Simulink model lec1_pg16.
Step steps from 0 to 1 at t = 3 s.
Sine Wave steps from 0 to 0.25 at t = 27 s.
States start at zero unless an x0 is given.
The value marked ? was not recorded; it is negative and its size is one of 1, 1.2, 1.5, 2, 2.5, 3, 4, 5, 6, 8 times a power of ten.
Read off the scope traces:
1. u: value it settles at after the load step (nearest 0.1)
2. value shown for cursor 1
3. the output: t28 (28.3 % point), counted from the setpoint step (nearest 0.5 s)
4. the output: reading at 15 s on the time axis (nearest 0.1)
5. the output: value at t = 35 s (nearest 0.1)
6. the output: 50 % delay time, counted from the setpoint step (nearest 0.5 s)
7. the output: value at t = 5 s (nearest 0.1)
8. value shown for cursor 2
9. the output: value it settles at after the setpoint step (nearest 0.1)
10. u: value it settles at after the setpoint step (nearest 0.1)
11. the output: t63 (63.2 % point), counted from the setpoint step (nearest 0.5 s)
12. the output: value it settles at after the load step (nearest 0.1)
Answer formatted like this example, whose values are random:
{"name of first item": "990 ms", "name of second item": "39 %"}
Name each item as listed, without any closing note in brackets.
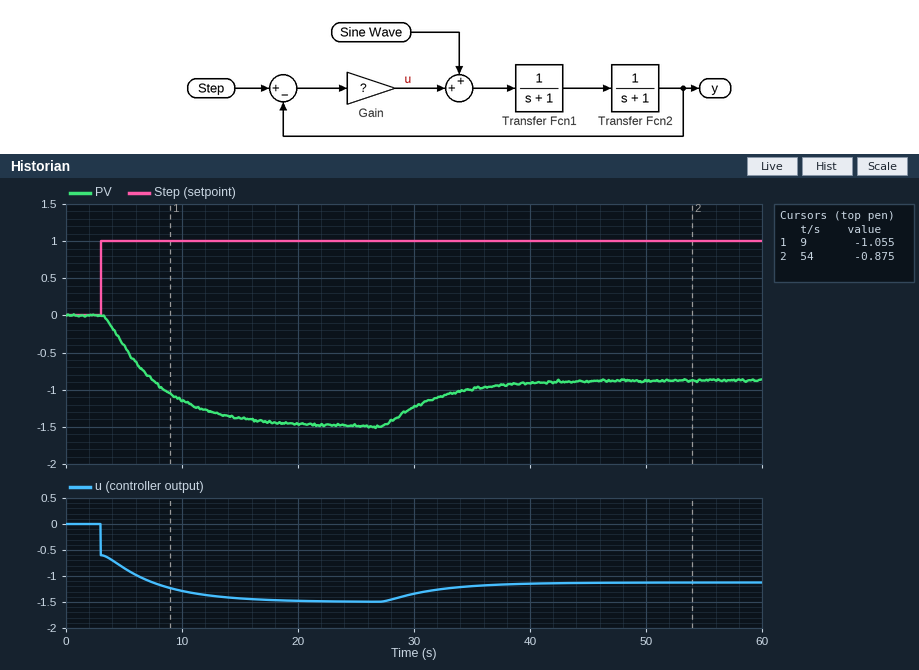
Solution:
{"u: value it settles at after the load step": "-1.1", "value shown for cursor 1": "-1.055", "the output: t28 (28.3 % point), counted from the setpoint step": "2.0 s", "the output: reading at 15 s on the time axis": "-1.4", "the output: value at t = 35 s": "-1.0", "the output: 50 % delay time, counted from the setpoint step": "3.5 s", "the output: value at t = 5 s": "-0.4", "value shown for cursor 2": "-0.875", "the output: value it settles at after the setpoint step": "-1.5", "u: value it settles at after the setpoint step": "-1.5", "the output: t63 (63.2 % point), counted from the setpoint step": "5.0 s", "the output: value it settles at after the load step": "-0.9"}
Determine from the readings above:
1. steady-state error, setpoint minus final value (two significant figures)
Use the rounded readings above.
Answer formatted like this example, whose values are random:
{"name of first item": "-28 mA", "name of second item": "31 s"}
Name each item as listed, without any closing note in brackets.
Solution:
{"steady-state error, setpoint minus final value": "2.5"}
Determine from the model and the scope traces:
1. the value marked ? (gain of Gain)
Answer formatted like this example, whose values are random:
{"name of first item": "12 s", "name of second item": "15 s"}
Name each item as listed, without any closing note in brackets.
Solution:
{"the value marked ?": "-0.6"}
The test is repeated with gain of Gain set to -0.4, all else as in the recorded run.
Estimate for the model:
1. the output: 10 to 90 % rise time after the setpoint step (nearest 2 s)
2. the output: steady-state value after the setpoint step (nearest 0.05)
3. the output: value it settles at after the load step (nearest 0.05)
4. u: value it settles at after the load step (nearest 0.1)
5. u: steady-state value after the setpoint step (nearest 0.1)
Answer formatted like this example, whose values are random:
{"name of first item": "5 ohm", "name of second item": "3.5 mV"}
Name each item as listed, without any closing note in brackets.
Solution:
{"the output: 10 to 90 % rise time after the setpoint step": "6 s", "the output: steady-state value after the setpoint step": "-0.65", "the output: value it settles at after the load step": "-0.25", "u: value it settles at after the load step": "-0.5", "u: steady-state value after the setpoint step": "-0.7"}
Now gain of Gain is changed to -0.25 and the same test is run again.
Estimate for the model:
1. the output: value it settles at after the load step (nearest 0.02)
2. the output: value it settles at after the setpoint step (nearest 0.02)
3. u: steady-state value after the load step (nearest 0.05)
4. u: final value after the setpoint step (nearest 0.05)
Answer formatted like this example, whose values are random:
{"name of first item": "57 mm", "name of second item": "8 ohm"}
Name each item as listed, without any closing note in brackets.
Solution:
{"the output: value it settles at after the load step": "0.00", "the output: value it settles at after the setpoint step": "-0.34", "u: steady-state value after the load step": "-0.25", "u: final value after the setpoint step": "-0.35"}
